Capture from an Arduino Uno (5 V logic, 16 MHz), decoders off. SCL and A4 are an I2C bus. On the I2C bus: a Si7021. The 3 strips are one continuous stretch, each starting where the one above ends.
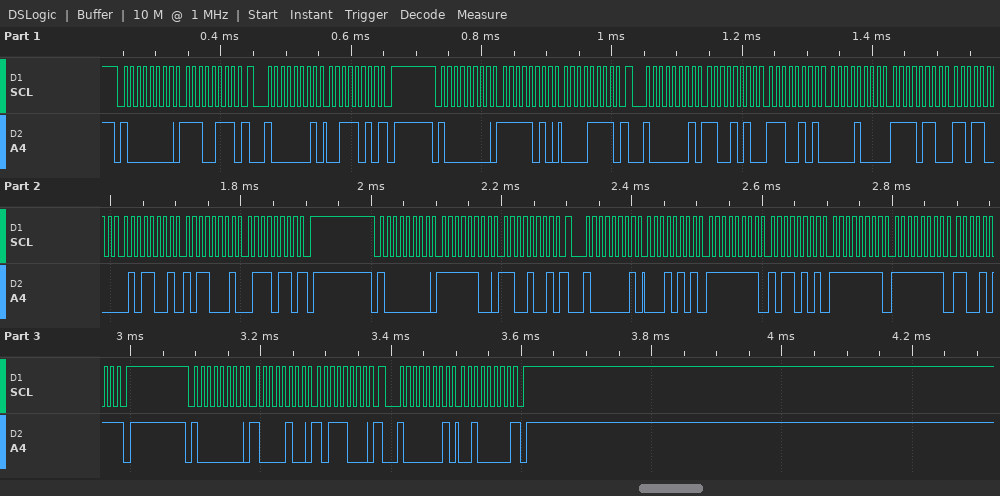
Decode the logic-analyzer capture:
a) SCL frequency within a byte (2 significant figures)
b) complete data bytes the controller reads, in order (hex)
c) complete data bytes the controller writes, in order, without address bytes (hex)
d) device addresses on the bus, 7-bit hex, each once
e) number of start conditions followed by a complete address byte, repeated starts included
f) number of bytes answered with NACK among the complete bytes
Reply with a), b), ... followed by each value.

a) 100 kHz
b) 3A CA E5 08 F6 D8 59 B1 76 15 FF B5 FF FF CB 20
c) E7 FA 0F FC C9 84 B8
d) 0x40
e) 8
f) 4
